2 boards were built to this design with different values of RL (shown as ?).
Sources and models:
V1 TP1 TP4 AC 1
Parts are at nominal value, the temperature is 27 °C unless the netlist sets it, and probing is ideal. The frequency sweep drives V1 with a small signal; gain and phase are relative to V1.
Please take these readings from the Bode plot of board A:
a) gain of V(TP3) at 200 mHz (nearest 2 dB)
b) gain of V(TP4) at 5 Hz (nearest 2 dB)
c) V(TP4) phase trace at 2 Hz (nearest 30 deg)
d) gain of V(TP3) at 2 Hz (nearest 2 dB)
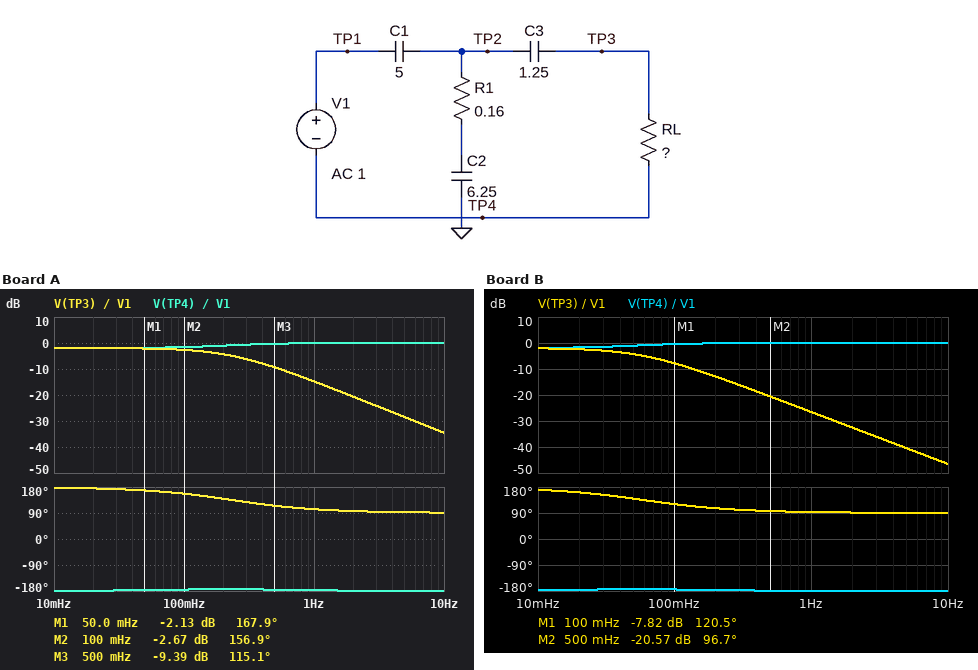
-4 dB
0 dB
-180 deg
-20 dB
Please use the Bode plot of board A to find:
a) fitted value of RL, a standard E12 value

0.68 Ω
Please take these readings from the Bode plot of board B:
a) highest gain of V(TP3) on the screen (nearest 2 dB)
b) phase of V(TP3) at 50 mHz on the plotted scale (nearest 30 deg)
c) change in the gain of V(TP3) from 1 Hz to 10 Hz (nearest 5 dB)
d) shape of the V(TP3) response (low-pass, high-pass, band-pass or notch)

-2 dB
150 deg
-20 dB
low-pass
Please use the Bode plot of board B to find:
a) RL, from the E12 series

2.7 Ω
